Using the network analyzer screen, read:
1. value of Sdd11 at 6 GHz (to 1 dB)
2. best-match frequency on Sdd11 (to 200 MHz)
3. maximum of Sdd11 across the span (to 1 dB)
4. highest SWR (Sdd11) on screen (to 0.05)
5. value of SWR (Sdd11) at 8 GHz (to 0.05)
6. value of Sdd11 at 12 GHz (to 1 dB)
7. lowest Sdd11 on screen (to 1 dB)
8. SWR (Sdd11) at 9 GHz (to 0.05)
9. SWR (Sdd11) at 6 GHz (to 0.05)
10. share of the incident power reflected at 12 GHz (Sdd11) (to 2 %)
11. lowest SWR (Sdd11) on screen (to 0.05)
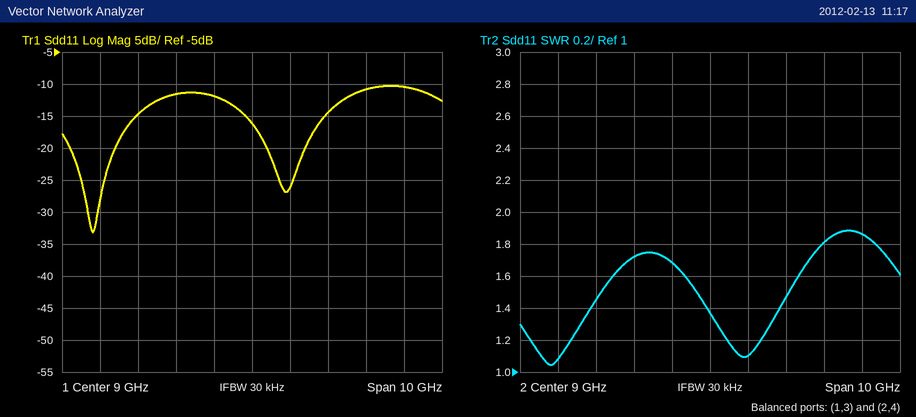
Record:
-15 dB
4.8 GHz
-10 dB
1.90
1.70
-11 dB
-33 dB
1.35
1.45
8 %
1.05
